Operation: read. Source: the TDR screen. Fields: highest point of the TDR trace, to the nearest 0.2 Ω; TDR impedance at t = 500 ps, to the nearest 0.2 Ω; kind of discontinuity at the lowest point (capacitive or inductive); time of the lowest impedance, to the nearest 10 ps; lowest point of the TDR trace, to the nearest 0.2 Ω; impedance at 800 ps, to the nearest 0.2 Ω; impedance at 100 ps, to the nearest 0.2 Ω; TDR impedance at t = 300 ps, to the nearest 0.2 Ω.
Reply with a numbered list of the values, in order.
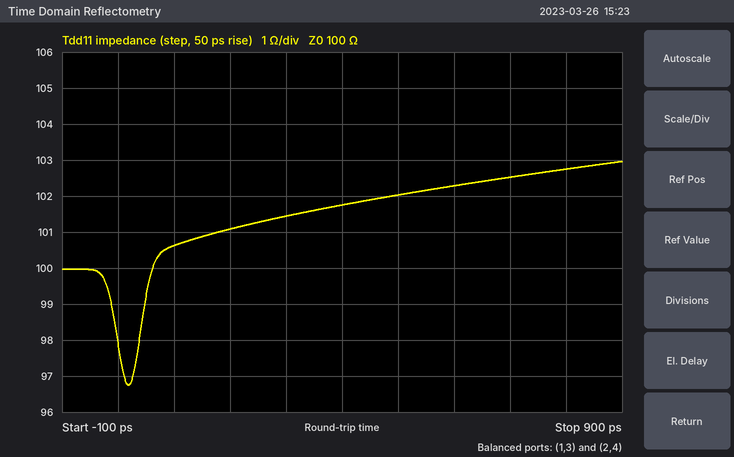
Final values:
1. 103.0 Ω
2. 102.0 Ω
3. capacitive
4. 20 ps
5. 96.8 Ω
6. 102.8 Ω
7. 100.6 Ω
8. 101.4 Ω
